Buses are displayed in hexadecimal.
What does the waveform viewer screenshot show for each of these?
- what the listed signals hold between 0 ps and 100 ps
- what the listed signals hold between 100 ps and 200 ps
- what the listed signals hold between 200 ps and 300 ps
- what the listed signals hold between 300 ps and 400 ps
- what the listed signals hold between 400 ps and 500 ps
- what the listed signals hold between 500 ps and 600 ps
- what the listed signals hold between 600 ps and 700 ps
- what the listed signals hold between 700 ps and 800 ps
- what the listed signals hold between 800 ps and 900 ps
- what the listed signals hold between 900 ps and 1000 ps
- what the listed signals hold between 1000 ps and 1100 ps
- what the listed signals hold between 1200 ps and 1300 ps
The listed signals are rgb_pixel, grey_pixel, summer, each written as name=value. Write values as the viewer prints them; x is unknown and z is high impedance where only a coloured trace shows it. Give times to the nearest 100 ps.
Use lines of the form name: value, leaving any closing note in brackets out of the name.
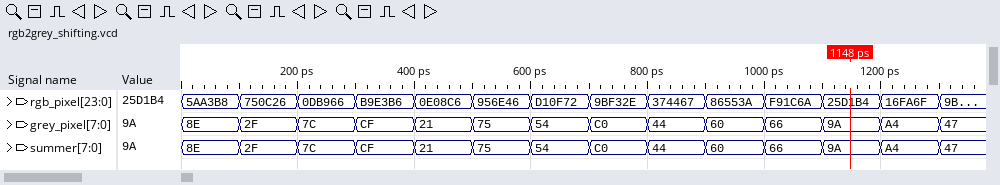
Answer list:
what the listed signals hold between 0 ps and 100 ps: rgb_pixel=5AA3B8, grey_pixel=8E, summer=8E
what the listed signals hold between 100 ps and 200 ps: rgb_pixel=750C26, grey_pixel=2F, summer=2F
what the listed signals hold between 200 ps and 300 ps: rgb_pixel=0DB966, grey_pixel=7C, summer=7C
what the listed signals hold between 300 ps and 400 ps: rgb_pixel=B9E3B6, grey_pixel=CF, summer=CF
what the listed signals hold between 400 ps and 500 ps: rgb_pixel=0E08C6, grey_pixel=21, summer=21
what the listed signals hold between 500 ps and 600 ps: rgb_pixel=956E46, grey_pixel=75, summer=75
what the listed signals hold between 600 ps and 700 ps: rgb_pixel=D10F72, grey_pixel=54, summer=54
what the listed signals hold between 700 ps and 800 ps: rgb_pixel=9BF32E, grey_pixel=C0, summer=C0
what the listed signals hold between 800 ps and 900 ps: rgb_pixel=374467, grey_pixel=44, summer=44
what the listed signals hold between 900 ps and 1000 ps: rgb_pixel=86553A, grey_pixel=60, summer=60
what the listed signals hold between 1000 ps and 1100 ps: rgb_pixel=F91C6A, grey_pixel=66, summer=66
what the listed signals hold between 1200 ps and 1300 ps: rgb_pixel=16FA6F, grey_pixel=A4, summer=A4
